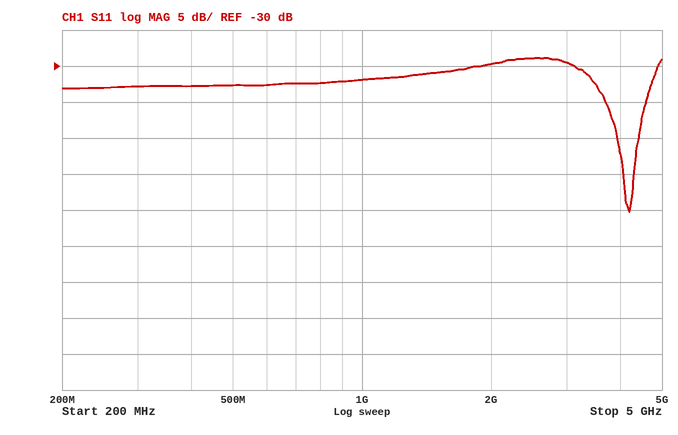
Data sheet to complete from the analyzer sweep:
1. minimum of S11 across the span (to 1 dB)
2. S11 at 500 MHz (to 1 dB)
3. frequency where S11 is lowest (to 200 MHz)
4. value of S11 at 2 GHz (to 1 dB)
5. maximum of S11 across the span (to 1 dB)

-50 dB
-33 dB
4.2 GHz
-30 dB
-29 dB
